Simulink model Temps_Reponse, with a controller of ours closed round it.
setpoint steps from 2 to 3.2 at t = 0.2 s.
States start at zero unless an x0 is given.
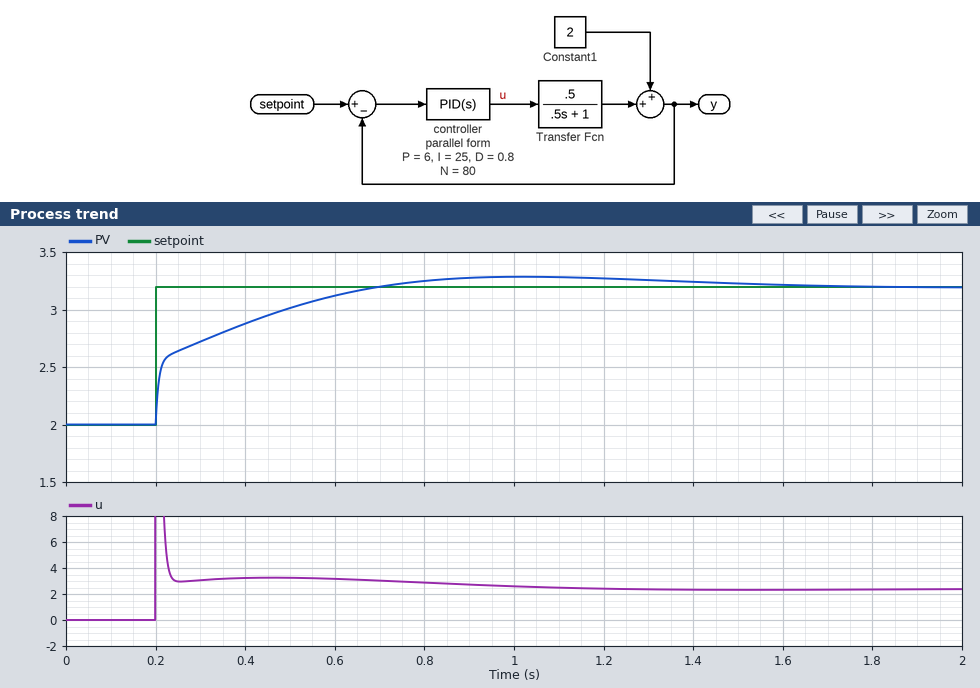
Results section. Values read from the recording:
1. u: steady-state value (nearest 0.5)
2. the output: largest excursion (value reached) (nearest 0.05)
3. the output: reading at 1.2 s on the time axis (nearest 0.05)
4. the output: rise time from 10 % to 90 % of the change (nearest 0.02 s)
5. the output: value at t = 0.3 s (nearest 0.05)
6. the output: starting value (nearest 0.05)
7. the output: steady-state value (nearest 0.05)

2.5
3.30
3.25
0.36 s
2.70
2.00
3.20
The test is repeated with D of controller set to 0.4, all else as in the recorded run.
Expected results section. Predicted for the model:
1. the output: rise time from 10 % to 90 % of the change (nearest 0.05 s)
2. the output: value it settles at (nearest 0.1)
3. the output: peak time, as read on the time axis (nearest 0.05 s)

0.30 s
3.2
0.90 s
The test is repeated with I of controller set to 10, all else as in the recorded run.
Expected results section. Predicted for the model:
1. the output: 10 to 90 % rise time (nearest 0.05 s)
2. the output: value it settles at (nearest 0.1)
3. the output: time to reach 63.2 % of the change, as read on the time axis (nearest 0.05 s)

0.65 s
3.2
0.35 s
